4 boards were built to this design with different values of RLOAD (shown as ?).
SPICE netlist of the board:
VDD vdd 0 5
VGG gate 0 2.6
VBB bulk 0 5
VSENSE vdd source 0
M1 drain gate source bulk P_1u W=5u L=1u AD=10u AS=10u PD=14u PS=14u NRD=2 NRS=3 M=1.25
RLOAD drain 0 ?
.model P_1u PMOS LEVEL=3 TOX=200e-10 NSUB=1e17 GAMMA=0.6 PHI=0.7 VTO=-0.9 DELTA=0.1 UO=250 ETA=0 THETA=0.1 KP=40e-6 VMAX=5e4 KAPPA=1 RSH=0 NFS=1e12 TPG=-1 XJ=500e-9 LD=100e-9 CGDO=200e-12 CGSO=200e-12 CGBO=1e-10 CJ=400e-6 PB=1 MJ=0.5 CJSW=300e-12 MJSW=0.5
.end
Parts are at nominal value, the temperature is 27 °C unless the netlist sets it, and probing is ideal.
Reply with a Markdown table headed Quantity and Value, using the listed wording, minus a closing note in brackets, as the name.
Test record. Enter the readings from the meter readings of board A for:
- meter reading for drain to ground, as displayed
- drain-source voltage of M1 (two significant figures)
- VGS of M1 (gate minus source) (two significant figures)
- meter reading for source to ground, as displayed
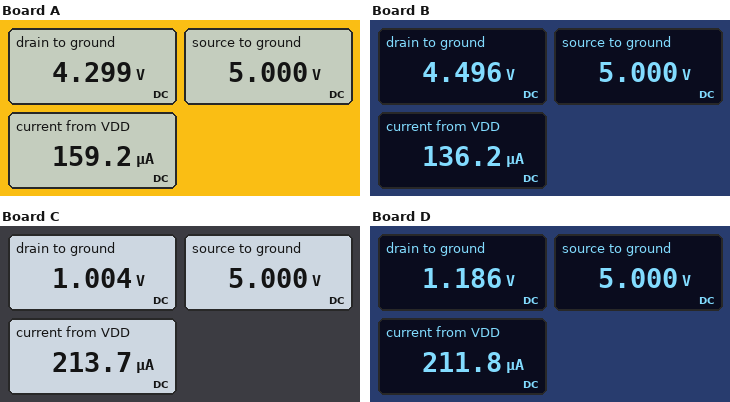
| Quantity | Value |
|---|---|
| meter reading for drain to ground, as displayed | 4.299 V |
| drain-source voltage of M1 | -700 mV |
| VGS of M1 (gate minus source) | -2.4 V |
| meter reading for source to ground, as displayed | 5.000 V |
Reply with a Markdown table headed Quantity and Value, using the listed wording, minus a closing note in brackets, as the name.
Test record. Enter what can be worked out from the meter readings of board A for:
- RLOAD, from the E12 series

| Quantity | Value |
|---|---|
| RLOAD, from the E12 series | 27 kΩ |
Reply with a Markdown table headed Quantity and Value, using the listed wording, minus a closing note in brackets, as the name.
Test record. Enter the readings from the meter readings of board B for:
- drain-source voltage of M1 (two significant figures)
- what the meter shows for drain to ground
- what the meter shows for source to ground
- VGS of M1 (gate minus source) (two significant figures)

| Quantity | Value |
|---|---|
| drain-source voltage of M1 | -500 mV |
| what the meter shows for drain to ground | 4.496 V |
| what the meter shows for source to ground | 5.000 V |
| VGS of M1 (gate minus source) | -2.4 V |
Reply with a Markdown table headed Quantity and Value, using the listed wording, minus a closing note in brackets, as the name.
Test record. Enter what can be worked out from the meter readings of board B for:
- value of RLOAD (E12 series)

| Quantity | Value |
|---|---|
| value of RLOAD | 33 kΩ |
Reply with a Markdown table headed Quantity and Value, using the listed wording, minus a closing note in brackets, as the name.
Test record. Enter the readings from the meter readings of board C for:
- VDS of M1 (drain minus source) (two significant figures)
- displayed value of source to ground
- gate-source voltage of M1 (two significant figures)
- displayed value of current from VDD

| Quantity | Value |
|---|---|
| VDS of M1 (drain minus source) | -4.0 V |
| displayed value of source to ground | 5.000 V |
| gate-source voltage of M1 | -2.4 V |
| displayed value of current from VDD | 213.7 µA |
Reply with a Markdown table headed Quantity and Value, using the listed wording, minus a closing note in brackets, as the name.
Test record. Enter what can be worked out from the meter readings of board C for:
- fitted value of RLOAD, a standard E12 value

| Quantity | Value |
|---|---|
| fitted value of RLOAD, a standard E12 value | 4.7 kΩ |
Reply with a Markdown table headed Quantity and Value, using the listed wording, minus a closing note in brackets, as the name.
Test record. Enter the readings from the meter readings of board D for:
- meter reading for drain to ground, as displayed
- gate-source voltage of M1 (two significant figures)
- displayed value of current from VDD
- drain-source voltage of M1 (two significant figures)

| Quantity | Value |
|---|---|
| meter reading for drain to ground, as displayed | 1.186 V |
| gate-source voltage of M1 | -2.4 V |
| displayed value of current from VDD | 211.8 µA |
| drain-source voltage of M1 | -3.8 V |
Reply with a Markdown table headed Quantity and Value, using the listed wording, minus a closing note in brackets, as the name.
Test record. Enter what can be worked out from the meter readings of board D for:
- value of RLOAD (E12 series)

| Quantity | Value |
|---|---|
| value of RLOAD | 5.6 kΩ |
